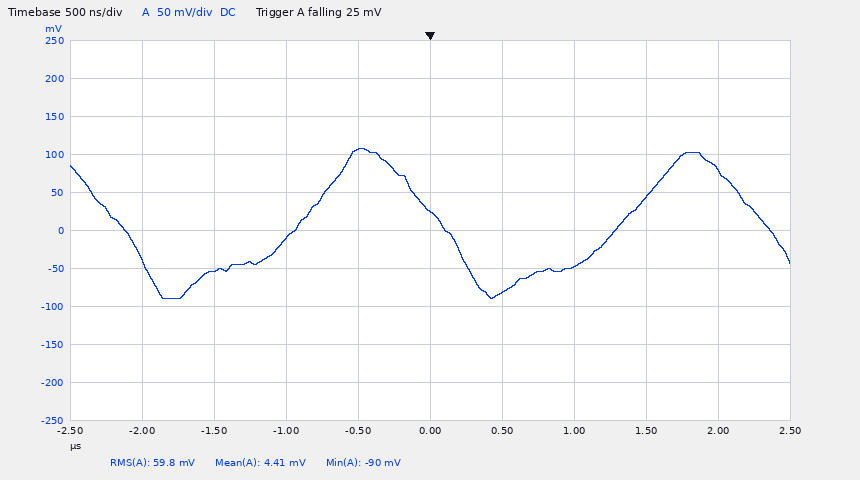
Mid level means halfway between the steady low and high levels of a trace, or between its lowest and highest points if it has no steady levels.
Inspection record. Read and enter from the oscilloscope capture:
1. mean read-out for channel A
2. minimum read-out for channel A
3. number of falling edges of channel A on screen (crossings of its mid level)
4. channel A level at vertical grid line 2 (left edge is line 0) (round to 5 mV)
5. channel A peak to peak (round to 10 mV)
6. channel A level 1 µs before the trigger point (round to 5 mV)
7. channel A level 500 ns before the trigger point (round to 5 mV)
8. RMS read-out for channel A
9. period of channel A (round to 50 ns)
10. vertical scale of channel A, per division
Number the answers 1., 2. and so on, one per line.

1. 4.41 mV
2. -90 mV
3. 3
4. -55 mV
5. 200 mV
6. -10 mV
7. 105 mV
8. 59.8 mV
9. 2.25 µs
10. 50 mV
